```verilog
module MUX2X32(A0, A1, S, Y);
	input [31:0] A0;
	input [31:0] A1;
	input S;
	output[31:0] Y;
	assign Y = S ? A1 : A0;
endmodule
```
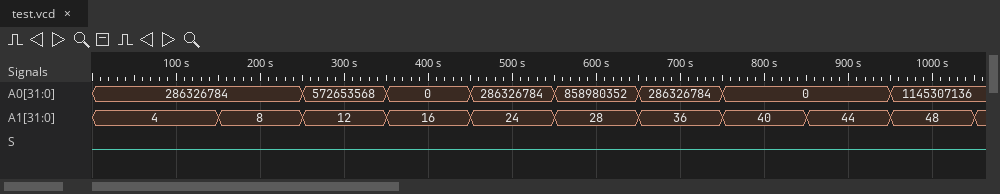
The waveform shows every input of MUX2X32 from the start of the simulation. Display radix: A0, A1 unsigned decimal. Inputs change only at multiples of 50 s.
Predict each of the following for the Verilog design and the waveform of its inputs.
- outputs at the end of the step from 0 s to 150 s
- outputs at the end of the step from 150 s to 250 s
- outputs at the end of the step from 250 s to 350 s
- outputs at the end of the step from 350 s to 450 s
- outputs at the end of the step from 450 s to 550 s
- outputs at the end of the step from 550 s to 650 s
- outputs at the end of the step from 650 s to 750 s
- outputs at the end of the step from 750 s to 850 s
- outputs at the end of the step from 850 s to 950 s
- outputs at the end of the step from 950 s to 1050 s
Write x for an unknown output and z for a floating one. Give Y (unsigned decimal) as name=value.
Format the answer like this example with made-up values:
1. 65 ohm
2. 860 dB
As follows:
1. Y=286326784
2. Y=286326784
3. Y=572653568
4. Y=0
5. Y=286326784
6. Y=858980352
7. Y=286326784
8. Y=0
9. Y=0
10. Y=1145307136
